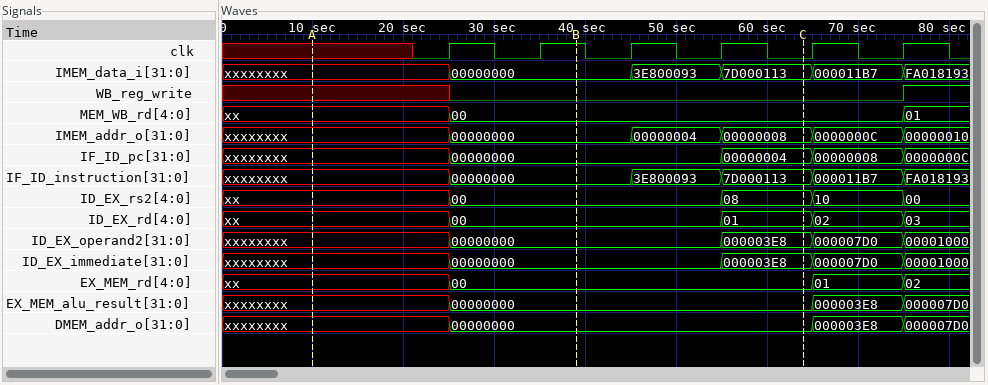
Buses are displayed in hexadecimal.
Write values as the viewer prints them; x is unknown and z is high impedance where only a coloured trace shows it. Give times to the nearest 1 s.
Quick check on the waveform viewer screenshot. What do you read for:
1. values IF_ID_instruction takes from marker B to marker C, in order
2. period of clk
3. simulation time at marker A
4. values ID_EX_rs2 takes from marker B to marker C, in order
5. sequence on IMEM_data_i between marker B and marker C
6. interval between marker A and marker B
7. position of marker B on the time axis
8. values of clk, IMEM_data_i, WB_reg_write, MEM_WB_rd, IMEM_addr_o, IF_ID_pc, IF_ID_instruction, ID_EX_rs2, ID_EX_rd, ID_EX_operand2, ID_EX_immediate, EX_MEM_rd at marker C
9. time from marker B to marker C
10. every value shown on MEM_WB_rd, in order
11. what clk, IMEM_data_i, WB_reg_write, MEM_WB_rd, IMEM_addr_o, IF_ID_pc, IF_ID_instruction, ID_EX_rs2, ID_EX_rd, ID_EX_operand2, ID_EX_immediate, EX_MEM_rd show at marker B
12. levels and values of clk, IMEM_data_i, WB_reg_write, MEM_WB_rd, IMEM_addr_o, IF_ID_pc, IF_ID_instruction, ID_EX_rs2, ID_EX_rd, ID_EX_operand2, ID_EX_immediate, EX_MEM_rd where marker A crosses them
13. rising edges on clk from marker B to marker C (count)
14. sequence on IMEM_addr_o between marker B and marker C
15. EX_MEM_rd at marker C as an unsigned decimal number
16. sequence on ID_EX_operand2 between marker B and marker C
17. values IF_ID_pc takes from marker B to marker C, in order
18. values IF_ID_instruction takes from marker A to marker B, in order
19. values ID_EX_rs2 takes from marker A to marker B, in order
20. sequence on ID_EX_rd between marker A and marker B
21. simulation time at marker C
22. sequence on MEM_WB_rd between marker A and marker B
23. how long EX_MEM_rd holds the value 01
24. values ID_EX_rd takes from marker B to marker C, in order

00000000, 3E800093, 7D000113
10 s
10 s
00, 08
00000000, 3E800093, 7D000113
29 s
39 s
clk=0, IMEM_data_i=7D000113, WB_reg_write=0, MEM_WB_rd=00, IMEM_addr_o=00000008, IF_ID_pc=00000004, IF_ID_instruction=7D000113, ID_EX_rs2=08, ID_EX_rd=01, ID_EX_operand2=000003E8, ID_EX_immediate=000003E8, EX_MEM_rd=00
25 s
xx, 00, 01
clk=1, IMEM_data_i=00000000, WB_reg_write=0, MEM_WB_rd=00, IMEM_addr_o=00000000, IF_ID_pc=00000000, IF_ID_instruction=00000000, ID_EX_rs2=00, ID_EX_rd=00, ID_EX_operand2=00000000, ID_EX_immediate=00000000, EX_MEM_rd=00
clk=x, IMEM_data_i=xxxxxxxx, WB_reg_write=x, MEM_WB_rd=xx, IMEM_addr_o=xxxxxxxx, IF_ID_pc=xxxxxxxx, IF_ID_instruction=xxxxxxxx, ID_EX_rs2=xx, ID_EX_rd=xx, ID_EX_operand2=xxxxxxxx, ID_EX_immediate=xxxxxxxx, EX_MEM_rd=xx
2
00000000, 00000004, 00000008
0
00000000, 000003E8
00000000, 00000004
xxxxxxxx, 00000000
xx, 00
xx, 00
64 s
xx, 00
10 s
00, 01
